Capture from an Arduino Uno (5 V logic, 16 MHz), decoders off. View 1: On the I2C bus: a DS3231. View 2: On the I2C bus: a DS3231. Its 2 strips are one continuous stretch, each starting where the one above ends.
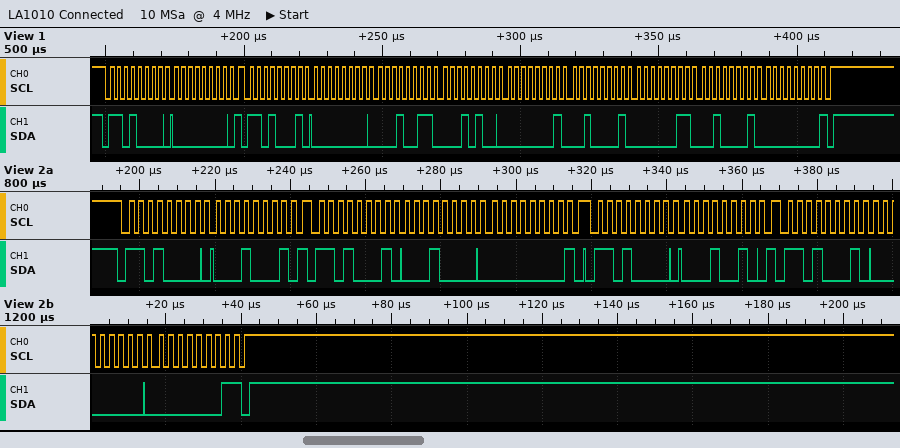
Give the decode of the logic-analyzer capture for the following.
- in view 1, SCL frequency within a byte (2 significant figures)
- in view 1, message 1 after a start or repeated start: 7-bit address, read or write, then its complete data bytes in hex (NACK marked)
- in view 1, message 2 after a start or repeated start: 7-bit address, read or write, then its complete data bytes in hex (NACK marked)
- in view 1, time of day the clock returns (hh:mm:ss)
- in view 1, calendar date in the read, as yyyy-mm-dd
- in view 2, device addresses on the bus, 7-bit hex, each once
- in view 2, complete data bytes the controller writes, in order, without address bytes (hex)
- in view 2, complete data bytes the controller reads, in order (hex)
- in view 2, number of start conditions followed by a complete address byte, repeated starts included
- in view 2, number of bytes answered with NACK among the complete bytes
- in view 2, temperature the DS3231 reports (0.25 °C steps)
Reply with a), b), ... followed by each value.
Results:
a) 400 kHz
b) 0x68 write: 00
c) 0x68 read: 00 13 14 01 21 03 21 00 NACK
d) 14:13:00
e) 2021-03-21
f) 0x68
g) 11 12
h) 10 00 00 01
i) 4
j) 2
k) 16.00 °C
